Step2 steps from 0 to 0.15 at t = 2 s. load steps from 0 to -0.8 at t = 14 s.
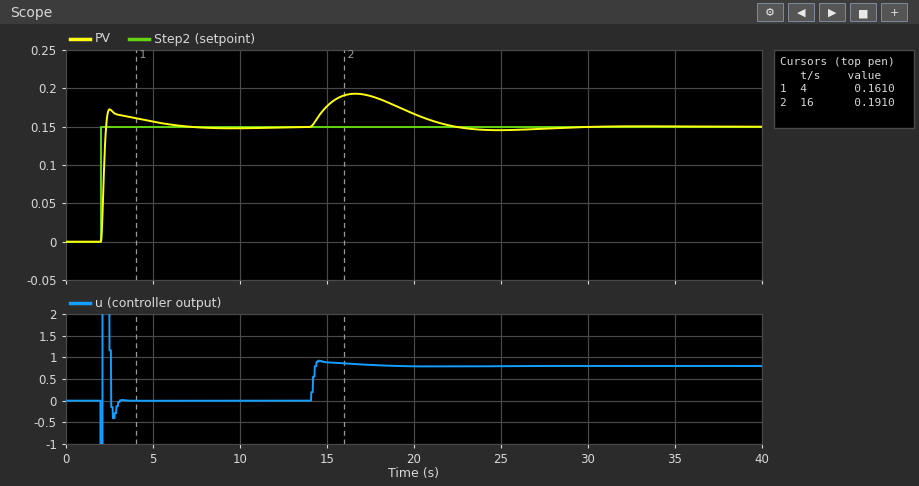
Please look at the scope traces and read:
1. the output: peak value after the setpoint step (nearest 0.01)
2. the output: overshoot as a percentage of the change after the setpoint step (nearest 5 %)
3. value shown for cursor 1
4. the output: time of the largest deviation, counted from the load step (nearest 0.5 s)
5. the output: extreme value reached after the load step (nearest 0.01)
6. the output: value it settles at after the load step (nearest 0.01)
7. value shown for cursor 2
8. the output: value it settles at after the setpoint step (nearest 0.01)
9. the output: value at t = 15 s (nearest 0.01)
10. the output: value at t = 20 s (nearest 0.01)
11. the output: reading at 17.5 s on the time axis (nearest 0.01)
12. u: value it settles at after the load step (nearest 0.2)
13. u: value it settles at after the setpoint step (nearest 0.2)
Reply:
0.17
15 %
0.1610
2.5 s
0.19
0.15
0.1910
0.15
0.18
0.17
0.19
0.8
0.0
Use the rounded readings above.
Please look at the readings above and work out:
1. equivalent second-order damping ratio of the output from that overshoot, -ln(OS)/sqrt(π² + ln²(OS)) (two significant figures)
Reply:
0.52
